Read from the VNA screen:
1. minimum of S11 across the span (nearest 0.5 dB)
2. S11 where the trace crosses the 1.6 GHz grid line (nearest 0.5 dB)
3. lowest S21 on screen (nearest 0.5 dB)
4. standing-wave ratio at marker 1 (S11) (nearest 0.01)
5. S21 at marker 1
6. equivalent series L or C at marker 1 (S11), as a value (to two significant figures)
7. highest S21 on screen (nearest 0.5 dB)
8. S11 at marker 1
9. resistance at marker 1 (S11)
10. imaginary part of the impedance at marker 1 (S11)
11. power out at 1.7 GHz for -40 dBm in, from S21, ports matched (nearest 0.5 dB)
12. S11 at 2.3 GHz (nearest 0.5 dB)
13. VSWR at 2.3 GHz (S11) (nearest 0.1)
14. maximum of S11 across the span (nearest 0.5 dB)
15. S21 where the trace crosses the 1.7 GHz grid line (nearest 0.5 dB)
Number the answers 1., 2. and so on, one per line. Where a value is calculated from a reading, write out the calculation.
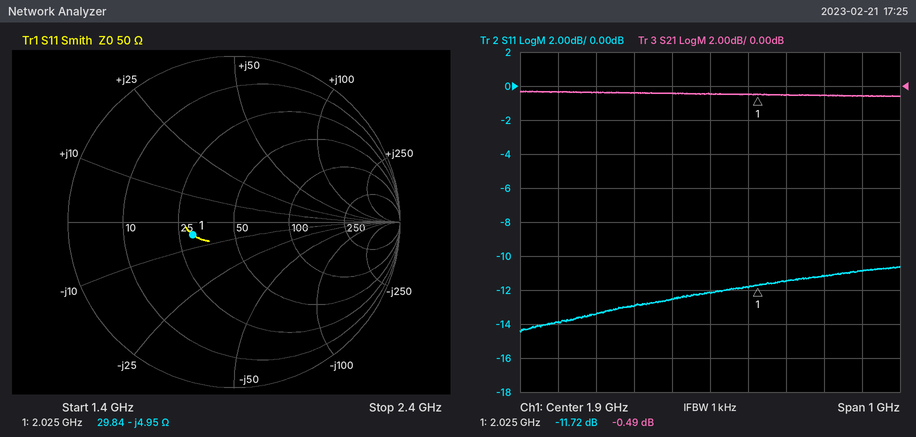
1. -14.5 dB
2. -13.5 dB
3. -0.5 dB
4. 1.70
5. -0.49 dB
6. C = 1/(2π × 2.025 GHz × 4.95 Ω) ≈ 16 pF
7. -0.5 dB
8. -11.72 dB
9. 29.84 Ω
10. -4.95 Ω
11. -40 dBm + (-0.5 dB) = -40.5 dBm
12. -11.0 dB
13. |Γ| = 10^(-11/20) = 0.2818; VSWR = (1 + 0.2818)/(1 − 0.2818) ≈ 1.8
14. -10.5 dB
15. -0.5 dB
